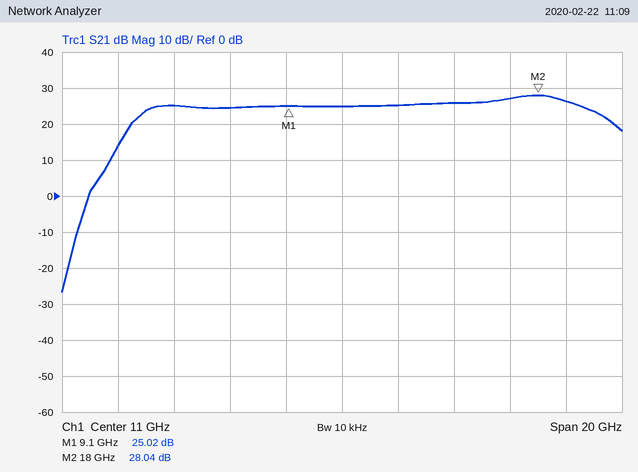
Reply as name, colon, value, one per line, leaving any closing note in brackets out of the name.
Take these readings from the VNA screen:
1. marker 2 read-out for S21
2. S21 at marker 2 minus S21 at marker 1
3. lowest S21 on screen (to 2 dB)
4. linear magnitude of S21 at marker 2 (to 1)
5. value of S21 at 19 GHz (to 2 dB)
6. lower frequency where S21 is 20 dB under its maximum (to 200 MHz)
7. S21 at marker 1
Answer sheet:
marker 2 read-out for S21: 28.04 dB
S21 at marker 2 minus S21 at marker 1: 3.02 dB
lowest S21 on screen: -26 dB
linear magnitude of S21 at marker 2: 25
value of S21 at 19 GHz: 26 dB
lower frequency where S21 is 20 dB under its maximum: 2.6 GHz
S21 at marker 1: 25.02 dB
